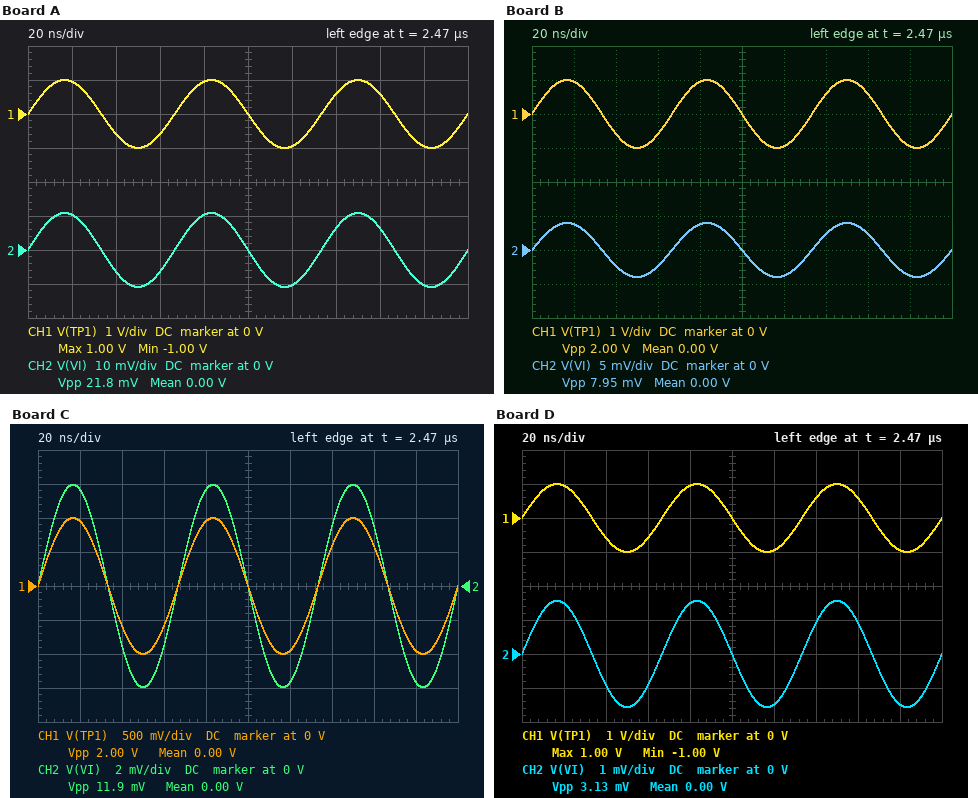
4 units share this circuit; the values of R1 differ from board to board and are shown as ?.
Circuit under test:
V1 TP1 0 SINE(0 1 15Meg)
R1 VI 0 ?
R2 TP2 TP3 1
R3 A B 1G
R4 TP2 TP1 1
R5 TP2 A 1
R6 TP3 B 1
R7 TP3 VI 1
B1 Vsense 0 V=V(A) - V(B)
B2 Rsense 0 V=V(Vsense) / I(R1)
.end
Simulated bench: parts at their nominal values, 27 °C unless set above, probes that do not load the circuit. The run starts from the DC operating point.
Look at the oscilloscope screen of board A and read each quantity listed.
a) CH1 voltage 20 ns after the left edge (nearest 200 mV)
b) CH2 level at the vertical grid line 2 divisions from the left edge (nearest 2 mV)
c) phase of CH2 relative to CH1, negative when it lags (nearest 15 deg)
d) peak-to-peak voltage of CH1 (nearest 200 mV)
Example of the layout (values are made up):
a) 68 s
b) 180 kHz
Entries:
a) 1.0 V
b) -6 mV
c) 0 deg
d) 2.0 V
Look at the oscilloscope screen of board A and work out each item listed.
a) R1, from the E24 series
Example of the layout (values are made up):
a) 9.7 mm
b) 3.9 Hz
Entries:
a) 0.033 Ω
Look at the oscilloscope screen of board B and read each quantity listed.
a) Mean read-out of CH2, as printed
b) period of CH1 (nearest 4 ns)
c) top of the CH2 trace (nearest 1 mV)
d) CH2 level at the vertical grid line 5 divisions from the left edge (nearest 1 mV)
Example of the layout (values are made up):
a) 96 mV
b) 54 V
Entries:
a) 0.00 V
b) 68 ns
c) 4 mV
d) 0 V
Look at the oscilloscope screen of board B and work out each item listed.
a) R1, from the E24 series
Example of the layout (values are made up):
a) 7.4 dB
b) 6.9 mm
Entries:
a) 0.012 Ω
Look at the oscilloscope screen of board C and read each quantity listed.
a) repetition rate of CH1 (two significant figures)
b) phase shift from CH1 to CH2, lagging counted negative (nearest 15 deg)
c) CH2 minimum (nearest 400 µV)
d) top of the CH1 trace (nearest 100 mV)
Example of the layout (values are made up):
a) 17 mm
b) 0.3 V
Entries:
a) 15 MHz
b) 0 deg
c) -6.0 mV
d) 1.0 V
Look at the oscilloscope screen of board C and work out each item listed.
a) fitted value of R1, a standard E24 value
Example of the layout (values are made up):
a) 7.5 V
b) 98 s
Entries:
a) 0.018 Ω
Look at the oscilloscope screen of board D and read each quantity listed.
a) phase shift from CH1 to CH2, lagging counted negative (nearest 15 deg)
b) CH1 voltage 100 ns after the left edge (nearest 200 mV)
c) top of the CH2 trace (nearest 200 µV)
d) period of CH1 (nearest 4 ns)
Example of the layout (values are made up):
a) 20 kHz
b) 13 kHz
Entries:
a) 0 deg
b) 0 V
c) 1.6 mV
d) 68 ns
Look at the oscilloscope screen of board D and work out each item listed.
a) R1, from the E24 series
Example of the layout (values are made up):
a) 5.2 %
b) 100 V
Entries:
a) 4.7 mΩ
